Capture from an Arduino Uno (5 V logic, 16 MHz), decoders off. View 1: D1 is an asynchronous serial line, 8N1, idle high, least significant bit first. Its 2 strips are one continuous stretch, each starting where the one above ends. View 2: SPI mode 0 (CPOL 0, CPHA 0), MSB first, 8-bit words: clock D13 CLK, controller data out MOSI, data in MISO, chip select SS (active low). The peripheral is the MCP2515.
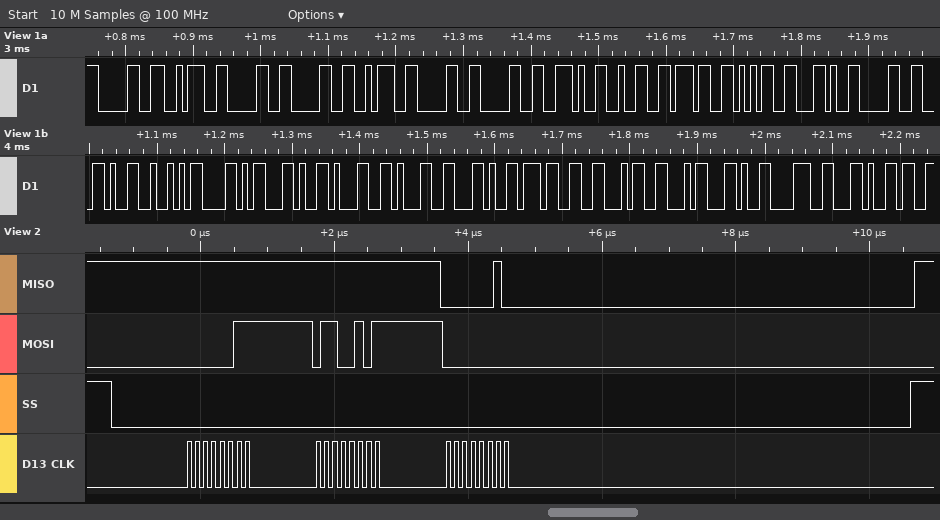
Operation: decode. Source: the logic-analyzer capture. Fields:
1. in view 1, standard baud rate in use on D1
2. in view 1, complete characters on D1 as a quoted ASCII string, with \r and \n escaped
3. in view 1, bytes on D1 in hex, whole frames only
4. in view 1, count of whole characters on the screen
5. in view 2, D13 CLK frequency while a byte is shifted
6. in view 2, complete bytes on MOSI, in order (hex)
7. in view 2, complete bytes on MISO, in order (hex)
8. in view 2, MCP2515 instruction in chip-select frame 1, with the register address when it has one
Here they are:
115200 baud
"0:00:00.275,0,RX,11,7FF,8,"
30 3A 30 30 3A 30 30 2E 32 37 35 2C 30 2C 52 58 2C 31 31 2C 37 46 46 2C 38 2C
26
8 MHz
03 65 00
FF FF 02
READ 0x65
